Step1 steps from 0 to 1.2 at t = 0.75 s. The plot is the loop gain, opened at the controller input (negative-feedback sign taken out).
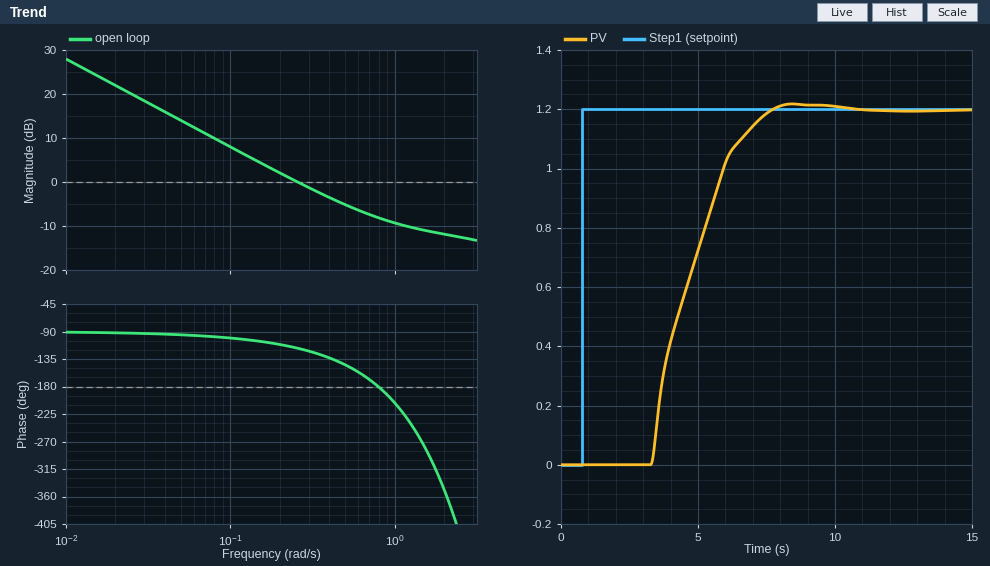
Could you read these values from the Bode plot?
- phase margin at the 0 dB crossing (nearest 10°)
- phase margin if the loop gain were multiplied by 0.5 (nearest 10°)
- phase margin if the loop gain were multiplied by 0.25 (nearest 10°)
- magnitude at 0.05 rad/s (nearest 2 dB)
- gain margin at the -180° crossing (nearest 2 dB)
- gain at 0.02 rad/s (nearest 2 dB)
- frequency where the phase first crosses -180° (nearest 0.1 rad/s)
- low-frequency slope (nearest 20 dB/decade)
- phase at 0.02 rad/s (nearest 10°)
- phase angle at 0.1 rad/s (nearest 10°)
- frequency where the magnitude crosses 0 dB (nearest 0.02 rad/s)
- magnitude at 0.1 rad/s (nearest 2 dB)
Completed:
60°
80°
80°
14 dB
8 dB
22 dB
0.8 rad/s
-20 dB/decade
-90°
-100°
0.26 rad/s
8 dB
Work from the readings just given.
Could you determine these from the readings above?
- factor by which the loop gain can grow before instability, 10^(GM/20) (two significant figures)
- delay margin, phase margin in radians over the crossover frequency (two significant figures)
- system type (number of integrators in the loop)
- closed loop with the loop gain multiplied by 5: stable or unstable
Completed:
2.5
4.0 s
1
unstable
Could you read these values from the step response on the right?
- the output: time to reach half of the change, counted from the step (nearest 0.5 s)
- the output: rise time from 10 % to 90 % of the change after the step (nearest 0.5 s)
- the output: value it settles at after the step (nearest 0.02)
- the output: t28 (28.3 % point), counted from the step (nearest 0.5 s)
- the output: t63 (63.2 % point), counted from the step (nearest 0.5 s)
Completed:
4.0 s
3.0 s
1.20
3.0 s
4.5 s
